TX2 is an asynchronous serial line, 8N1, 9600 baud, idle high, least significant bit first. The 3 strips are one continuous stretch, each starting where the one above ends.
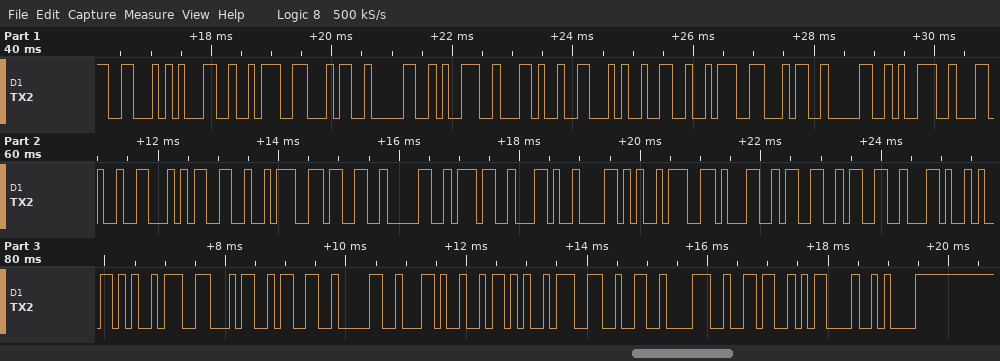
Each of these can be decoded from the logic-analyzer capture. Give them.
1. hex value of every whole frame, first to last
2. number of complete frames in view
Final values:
46 31 3A 34 30 39 2C 46 32 3A 34 30 39 2C 46 33 3A 33 30 37 2C 58 3A 31 33 33 2C 59 3A 34 33 30 2C 5A 3A 32 38 36 0D 0A
40
